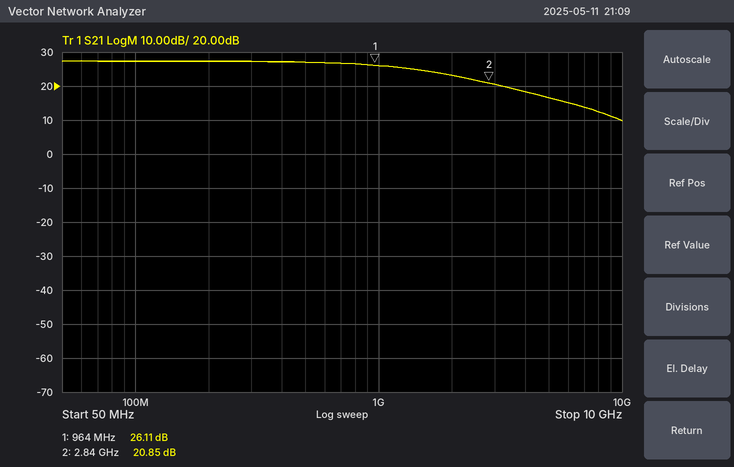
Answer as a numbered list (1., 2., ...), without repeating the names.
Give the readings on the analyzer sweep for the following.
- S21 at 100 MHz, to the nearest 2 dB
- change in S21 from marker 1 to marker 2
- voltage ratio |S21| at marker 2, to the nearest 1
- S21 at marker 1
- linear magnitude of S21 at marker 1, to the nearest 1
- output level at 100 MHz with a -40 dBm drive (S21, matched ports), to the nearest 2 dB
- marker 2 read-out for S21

1. 28 dB
2. -5.26 dB
3. 11
4. 26.11 dB
5. 20
6. -12 dBm
7. 20.85 dB
